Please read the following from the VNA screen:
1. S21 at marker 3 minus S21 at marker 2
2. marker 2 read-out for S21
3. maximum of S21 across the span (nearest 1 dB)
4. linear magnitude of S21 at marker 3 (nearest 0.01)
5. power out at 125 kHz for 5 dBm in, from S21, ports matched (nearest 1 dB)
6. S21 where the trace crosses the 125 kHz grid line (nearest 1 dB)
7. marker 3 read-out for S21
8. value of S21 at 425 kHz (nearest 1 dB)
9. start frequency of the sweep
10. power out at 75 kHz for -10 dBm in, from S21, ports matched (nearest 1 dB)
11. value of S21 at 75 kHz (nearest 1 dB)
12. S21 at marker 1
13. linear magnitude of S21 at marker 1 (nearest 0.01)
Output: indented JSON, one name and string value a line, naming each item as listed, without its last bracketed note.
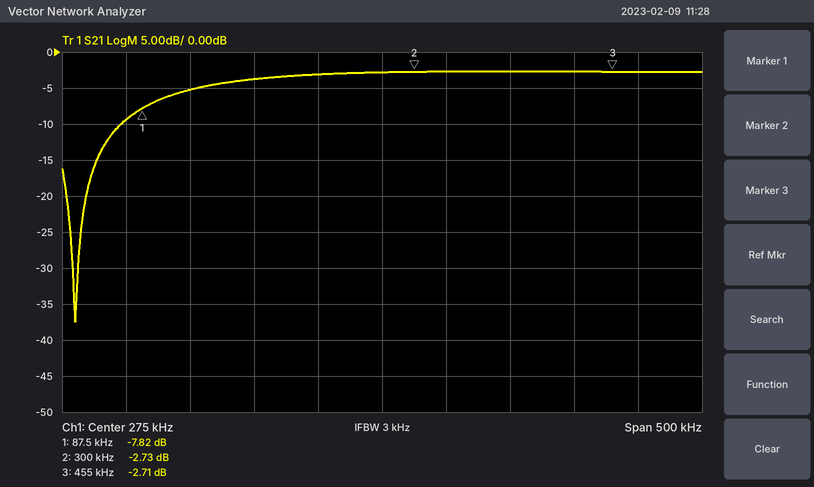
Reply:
{
  "S21 at marker 3 minus S21 at marker 2": "0.02 dB",
  "marker 2 read-out for S21": "-2.73 dB",
  "maximum of S21 across the span": "-3 dB",
  "linear magnitude of S21 at marker 3": "0.73",
  "power out at 125 kHz for 5 dBm in, from S21, ports matched": "0 dBm",
  "S21 where the trace crosses the 125 kHz grid line": "-5 dB",
  "marker 3 read-out for S21": "-2.71 dB",
  "value of S21 at 425 kHz": "-3 dB",
  "start frequency of the sweep": "25 kHz",
  "power out at 75 kHz for -10 dBm in, from S21, ports matched": "-19 dBm",
  "value of S21 at 75 kHz": "-9 dB",
  "S21 at marker 1": "-7.82 dB",
  "linear magnitude of S21 at marker 1": "0.41"
}
